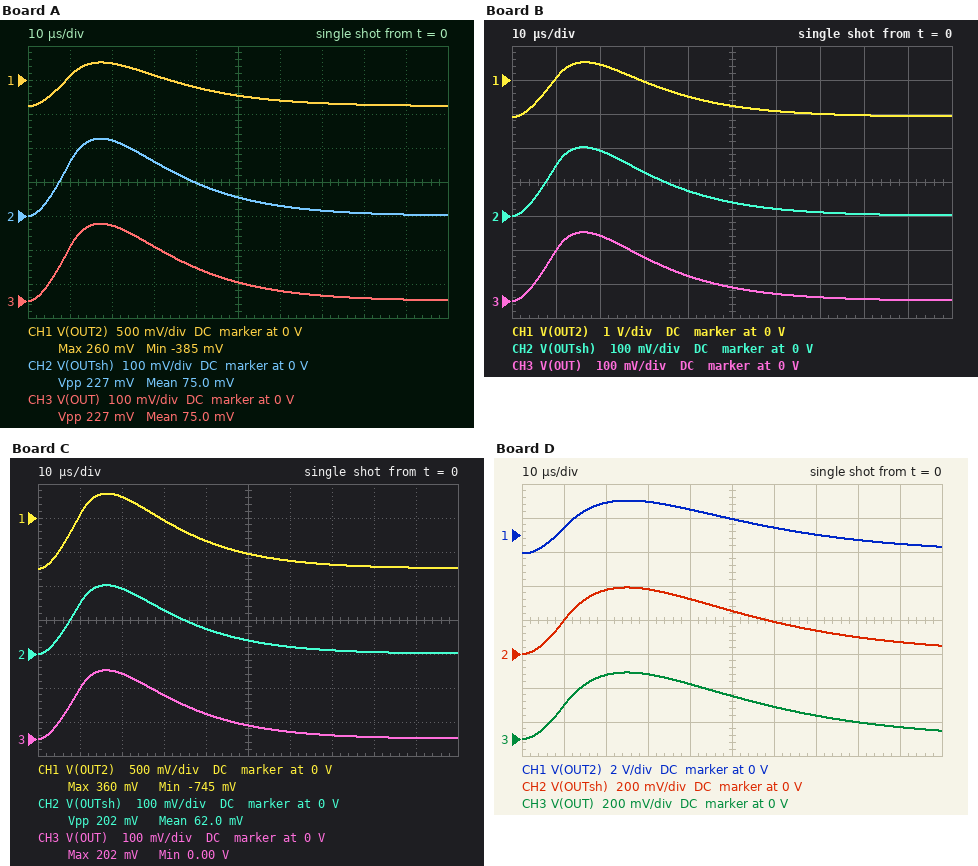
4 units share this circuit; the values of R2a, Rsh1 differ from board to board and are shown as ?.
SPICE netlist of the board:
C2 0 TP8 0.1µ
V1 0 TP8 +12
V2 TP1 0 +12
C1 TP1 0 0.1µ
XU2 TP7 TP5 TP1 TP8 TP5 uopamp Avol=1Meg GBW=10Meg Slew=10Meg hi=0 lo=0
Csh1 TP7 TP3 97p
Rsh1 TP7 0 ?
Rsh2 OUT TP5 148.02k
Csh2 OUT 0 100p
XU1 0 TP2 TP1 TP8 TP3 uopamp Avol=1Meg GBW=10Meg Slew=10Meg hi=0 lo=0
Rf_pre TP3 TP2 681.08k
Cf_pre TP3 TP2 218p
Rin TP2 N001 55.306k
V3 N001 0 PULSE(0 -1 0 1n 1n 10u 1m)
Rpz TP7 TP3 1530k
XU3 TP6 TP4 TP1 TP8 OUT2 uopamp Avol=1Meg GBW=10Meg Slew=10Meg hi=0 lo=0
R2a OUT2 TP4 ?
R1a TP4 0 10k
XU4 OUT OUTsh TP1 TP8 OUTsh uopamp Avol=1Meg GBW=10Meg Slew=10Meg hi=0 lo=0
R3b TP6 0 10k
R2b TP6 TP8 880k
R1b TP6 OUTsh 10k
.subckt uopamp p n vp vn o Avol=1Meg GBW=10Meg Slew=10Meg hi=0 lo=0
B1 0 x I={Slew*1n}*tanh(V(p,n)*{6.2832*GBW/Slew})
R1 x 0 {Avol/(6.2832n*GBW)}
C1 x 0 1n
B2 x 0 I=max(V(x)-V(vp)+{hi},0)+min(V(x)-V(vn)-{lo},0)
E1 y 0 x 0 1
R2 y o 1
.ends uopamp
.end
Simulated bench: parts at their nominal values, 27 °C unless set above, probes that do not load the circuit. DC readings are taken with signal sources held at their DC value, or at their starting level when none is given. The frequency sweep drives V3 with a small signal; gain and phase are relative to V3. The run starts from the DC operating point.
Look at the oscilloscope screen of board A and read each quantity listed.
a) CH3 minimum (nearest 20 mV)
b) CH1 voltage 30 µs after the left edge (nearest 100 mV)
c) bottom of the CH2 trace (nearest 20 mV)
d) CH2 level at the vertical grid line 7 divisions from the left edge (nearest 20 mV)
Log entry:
0 V
100 mV
0 V
20 mV
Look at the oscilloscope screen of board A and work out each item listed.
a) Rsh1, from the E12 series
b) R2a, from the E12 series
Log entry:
100 kΩ
47 kΩ
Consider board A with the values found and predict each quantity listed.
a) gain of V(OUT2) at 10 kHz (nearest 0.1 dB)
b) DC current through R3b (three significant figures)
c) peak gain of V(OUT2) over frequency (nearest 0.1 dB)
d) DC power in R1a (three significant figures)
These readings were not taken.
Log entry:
2.7 dB
6.78 µA
6.6 dB
460 nW
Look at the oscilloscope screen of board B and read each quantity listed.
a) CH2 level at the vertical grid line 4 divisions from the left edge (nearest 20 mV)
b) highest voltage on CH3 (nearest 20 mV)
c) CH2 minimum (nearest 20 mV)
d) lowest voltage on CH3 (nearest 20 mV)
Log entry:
80 mV
200 mV
0 V
0 V
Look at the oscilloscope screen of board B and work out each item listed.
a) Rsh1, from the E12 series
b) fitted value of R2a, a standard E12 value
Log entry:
82 kΩ
150 kΩ
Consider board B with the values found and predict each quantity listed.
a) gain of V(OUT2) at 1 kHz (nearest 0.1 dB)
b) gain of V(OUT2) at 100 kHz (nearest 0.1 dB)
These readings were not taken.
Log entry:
13.9 dB
-19.3 dB
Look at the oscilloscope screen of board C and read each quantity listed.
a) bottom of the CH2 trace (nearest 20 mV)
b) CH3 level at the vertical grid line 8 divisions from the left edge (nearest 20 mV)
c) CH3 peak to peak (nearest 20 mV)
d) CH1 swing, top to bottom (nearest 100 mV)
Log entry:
0 V
0 V
200 mV
1.1 V
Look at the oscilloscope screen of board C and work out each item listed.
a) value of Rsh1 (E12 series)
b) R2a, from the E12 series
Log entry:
82 kΩ
100 kΩ
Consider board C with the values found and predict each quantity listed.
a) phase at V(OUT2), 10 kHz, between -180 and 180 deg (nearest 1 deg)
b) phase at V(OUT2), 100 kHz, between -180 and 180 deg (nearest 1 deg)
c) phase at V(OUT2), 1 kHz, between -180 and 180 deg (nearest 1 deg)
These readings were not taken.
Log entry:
111 deg
10 deg
172 deg
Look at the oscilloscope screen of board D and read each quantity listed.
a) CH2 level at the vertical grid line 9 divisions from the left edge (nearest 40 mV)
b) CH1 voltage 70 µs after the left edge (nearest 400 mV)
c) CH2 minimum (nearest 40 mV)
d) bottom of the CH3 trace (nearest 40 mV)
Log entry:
80 mV
0 V
0 V
0 V
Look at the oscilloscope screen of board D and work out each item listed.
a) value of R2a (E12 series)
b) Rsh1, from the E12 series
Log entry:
150 kΩ
330 kΩ
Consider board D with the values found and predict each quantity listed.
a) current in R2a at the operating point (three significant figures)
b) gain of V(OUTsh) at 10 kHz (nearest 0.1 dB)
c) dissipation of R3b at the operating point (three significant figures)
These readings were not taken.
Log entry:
6.78 µA
-1.7 dB
460 nW
